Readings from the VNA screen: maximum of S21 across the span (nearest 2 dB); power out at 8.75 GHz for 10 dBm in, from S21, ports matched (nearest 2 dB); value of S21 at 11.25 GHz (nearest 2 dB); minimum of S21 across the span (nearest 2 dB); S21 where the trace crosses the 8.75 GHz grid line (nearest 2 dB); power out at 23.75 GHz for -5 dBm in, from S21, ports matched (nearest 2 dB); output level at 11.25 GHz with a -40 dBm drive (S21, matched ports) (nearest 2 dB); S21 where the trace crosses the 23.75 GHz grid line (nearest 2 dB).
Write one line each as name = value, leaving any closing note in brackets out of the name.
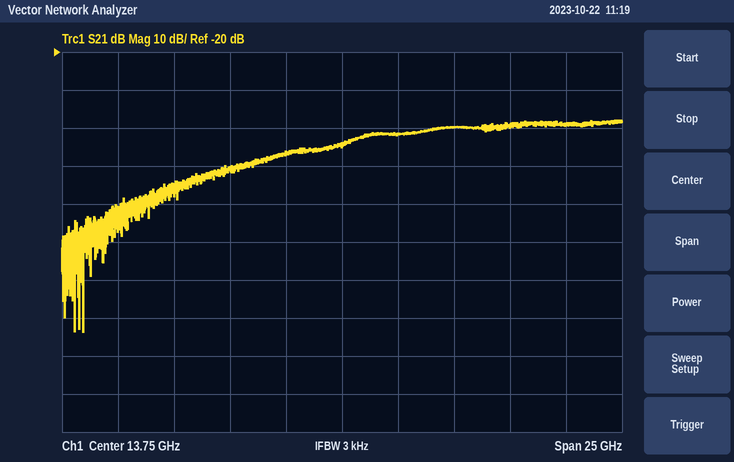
maximum of S21 across the span = -38 dB
power out at 8.75 GHz for 10 dBm in, from S21, ports matched = -40 dBm
value of S21 at 11.25 GHz = -46 dB
minimum of S21 across the span = -94 dB
S21 where the trace crosses the 8.75 GHz grid line = -50 dB
power out at 23.75 GHz for -5 dBm in, from S21, ports matched = -44 dBm
output level at 11.25 GHz with a -40 dBm drive (S21, matched ports) = -86 dBm
S21 where the trace crosses the 23.75 GHz grid line = -40 dB
